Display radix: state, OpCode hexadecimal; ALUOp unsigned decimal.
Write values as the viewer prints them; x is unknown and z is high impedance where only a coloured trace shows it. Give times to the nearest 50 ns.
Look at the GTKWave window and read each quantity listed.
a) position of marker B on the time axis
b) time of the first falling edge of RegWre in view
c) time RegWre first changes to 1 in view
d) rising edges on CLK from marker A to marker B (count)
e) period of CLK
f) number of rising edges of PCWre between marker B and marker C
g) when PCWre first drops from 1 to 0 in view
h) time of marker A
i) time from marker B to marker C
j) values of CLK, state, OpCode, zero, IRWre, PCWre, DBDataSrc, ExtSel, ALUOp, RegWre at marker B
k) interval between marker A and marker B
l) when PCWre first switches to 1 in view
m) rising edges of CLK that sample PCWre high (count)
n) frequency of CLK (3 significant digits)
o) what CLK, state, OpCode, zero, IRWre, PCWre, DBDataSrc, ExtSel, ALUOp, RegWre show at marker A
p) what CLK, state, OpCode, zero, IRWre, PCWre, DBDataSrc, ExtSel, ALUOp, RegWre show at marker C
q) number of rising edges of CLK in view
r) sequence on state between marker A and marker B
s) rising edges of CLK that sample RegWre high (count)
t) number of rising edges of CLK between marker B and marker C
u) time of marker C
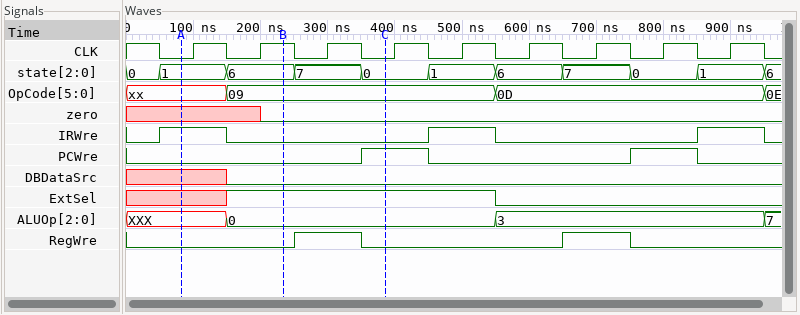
250 ns
350 ns
250 ns
2
100 ns
1
450 ns
100 ns
150 ns
CLK=1, state=6, OpCode=09, zero=0, IRWre=0, PCWre=0, DBDataSrc=0, ExtSel=1, ALUOp=0, RegWre=0
150 ns
350 ns
2
10.0 MHz
CLK=0, state=1, OpCode=xx, zero=x, IRWre=1, PCWre=0, DBDataSrc=x, ExtSel=x, ALUOp=XXX, RegWre=0
CLK=0, state=0, OpCode=09, zero=0, IRWre=0, PCWre=1, DBDataSrc=0, ExtSel=1, ALUOp=0, RegWre=0
9
1, 6
2
1
400 ns
